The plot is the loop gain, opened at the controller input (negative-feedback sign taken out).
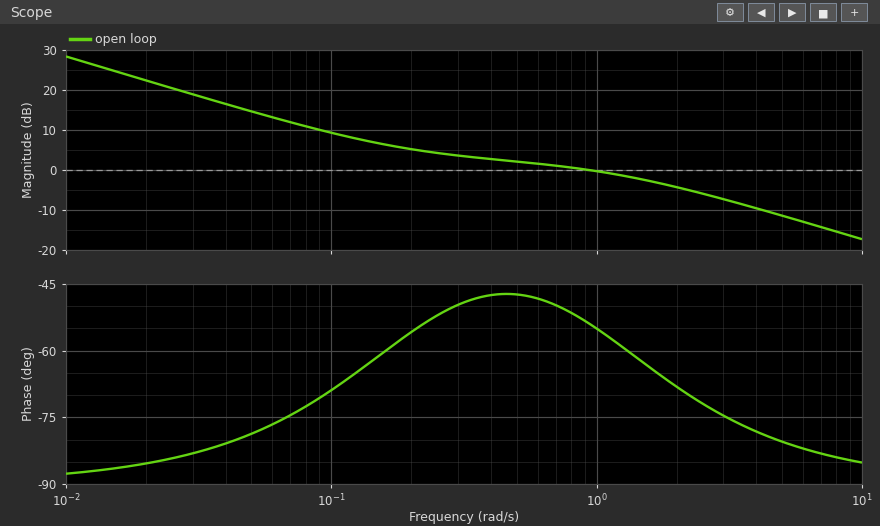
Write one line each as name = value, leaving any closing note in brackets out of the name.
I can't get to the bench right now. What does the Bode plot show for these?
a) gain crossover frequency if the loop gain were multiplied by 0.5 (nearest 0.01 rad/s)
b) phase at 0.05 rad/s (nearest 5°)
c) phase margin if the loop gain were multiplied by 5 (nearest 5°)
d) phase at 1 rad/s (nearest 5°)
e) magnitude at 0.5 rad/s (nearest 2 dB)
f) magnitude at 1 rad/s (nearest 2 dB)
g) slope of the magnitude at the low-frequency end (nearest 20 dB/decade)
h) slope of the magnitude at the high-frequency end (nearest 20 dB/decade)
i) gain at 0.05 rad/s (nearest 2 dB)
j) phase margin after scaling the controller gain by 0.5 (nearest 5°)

gain crossover frequency if the loop gain were multiplied by 0.5 = 0.17 rad/s
phase at 0.05 rad/s = -80°
phase margin if the loop gain were multiplied by 5 = 95°
phase at 1 rad/s = -55°
magnitude at 0.5 rad/s = 2 dB
magnitude at 1 rad/s = 0 dB
slope of the magnitude at the low-frequency end = -20 dB/decade
slope of the magnitude at the high-frequency end = -20 dB/decade
gain at 0.05 rad/s = 14 dB
phase margin after scaling the controller gain by 0.5 = 120°
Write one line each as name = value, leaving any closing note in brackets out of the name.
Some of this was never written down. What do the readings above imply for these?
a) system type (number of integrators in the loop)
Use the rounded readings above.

system type = 1
